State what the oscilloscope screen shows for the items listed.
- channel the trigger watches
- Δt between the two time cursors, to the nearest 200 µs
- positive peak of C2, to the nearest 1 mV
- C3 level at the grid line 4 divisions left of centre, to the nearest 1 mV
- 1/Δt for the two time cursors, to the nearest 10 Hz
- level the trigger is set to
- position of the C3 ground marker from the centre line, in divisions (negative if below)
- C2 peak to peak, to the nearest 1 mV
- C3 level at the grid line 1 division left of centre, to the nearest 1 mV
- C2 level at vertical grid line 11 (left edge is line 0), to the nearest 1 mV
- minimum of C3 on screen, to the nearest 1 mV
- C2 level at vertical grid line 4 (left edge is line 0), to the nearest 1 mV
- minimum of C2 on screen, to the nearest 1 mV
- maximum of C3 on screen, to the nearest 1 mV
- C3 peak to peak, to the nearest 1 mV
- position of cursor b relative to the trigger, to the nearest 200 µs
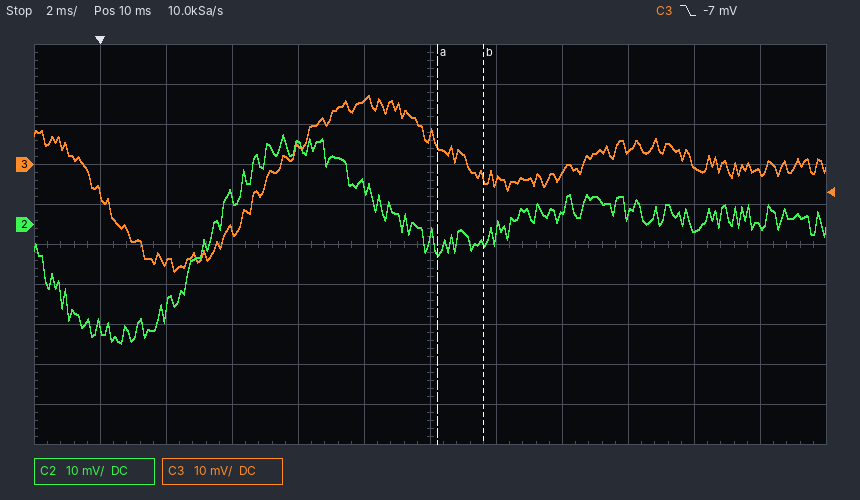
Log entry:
C3
1.4 ms
22 mV
-24 mV
710 Hz
-7 mV
+2.0 div
52 mV
16 mV
0 mV
-27 mV
20 mV
-30 mV
17 mV
44 mV
+11.6 ms
